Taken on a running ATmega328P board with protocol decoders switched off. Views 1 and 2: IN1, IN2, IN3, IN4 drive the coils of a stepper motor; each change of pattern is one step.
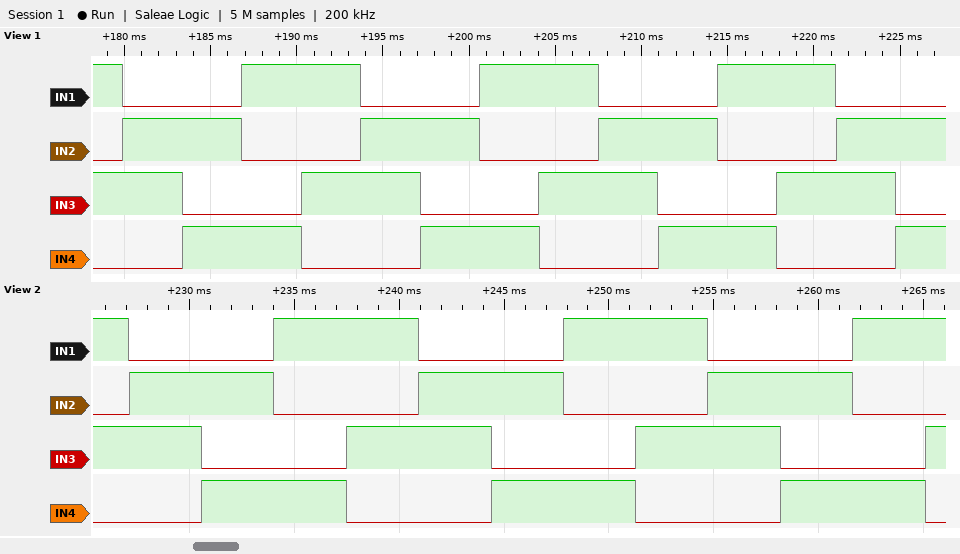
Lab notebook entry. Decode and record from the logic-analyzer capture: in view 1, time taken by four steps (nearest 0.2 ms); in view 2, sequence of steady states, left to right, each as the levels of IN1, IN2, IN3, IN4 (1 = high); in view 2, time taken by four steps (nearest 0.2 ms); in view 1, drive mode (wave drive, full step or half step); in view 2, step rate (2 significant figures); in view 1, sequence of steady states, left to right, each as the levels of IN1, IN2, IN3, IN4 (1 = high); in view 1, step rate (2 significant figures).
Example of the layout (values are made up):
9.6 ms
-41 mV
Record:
13.8 ms
1010 0110 0101 1001 1010 0110 0101 1001 1010 0110 0101 1001 1010
13.8 ms
full step
290 steps/s
1010 0110 0101 1001 1010 0110 0101 1001 1010 0110 0101 1001 1010 0110 0101
290 steps/s
